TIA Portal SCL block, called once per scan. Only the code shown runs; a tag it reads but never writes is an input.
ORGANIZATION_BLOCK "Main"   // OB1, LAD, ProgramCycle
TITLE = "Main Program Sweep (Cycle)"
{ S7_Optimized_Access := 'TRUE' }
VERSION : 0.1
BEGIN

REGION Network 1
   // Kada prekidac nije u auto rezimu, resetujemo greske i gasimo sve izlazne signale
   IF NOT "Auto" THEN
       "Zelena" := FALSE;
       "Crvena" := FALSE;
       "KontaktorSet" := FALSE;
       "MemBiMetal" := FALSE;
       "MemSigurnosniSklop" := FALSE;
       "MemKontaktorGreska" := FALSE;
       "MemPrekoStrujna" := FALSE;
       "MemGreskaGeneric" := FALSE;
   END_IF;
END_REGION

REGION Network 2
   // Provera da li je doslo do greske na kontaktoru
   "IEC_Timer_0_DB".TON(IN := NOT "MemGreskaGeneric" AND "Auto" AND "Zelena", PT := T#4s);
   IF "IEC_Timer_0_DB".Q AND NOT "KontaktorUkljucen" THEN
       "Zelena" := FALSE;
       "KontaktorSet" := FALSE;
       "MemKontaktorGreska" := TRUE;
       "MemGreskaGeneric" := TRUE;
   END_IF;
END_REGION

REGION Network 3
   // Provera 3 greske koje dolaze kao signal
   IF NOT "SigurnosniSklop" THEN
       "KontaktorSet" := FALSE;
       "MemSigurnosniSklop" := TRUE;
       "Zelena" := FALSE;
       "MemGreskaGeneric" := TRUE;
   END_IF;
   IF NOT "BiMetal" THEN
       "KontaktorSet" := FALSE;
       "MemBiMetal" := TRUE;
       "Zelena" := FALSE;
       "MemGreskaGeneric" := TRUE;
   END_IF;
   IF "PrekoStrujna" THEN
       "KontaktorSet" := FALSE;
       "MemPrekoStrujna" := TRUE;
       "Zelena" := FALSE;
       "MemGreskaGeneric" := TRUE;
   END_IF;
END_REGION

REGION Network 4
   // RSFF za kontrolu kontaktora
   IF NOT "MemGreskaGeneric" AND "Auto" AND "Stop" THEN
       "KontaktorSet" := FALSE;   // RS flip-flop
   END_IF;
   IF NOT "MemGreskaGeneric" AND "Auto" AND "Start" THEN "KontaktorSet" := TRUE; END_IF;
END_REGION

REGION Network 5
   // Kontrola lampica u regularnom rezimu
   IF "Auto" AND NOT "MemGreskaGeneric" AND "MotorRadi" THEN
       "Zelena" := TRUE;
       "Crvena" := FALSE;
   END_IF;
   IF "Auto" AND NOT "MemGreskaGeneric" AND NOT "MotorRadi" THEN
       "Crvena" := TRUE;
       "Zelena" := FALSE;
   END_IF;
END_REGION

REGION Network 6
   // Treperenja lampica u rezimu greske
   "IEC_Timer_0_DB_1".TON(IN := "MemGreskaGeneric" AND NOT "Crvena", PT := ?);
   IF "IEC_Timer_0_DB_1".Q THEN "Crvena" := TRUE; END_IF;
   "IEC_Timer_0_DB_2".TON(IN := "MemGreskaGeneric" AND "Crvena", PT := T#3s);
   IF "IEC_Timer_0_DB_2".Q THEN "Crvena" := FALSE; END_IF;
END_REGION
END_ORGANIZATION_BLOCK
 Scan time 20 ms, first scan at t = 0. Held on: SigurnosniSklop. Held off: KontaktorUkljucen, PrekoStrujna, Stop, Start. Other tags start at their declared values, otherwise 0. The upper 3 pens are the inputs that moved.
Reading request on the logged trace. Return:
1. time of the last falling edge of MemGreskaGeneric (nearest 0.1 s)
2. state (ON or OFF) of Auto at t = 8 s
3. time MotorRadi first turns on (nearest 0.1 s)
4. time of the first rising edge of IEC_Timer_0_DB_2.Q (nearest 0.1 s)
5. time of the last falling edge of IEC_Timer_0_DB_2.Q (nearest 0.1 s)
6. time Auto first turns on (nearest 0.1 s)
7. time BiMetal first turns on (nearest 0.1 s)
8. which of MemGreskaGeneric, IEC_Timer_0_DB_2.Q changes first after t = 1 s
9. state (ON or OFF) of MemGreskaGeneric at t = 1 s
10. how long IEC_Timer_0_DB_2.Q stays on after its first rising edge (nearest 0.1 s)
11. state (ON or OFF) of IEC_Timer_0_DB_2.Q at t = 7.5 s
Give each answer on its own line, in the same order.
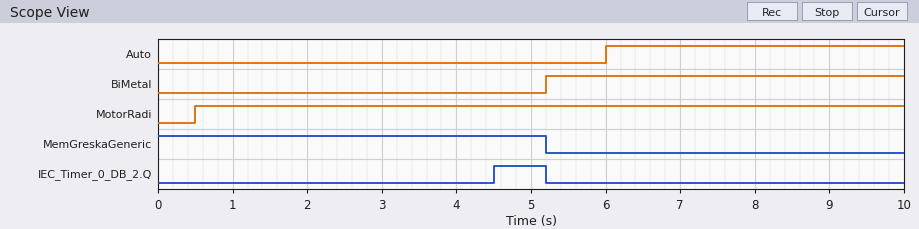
5.2 s
ON
0.5 s
4.5 s
5.2 s
6.0 s
5.2 s
IEC_Timer_0_DB_2.Q
ON
0.7 s
OFF
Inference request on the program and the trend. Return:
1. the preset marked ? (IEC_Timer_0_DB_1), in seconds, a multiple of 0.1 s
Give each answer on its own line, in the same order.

1.5 s
